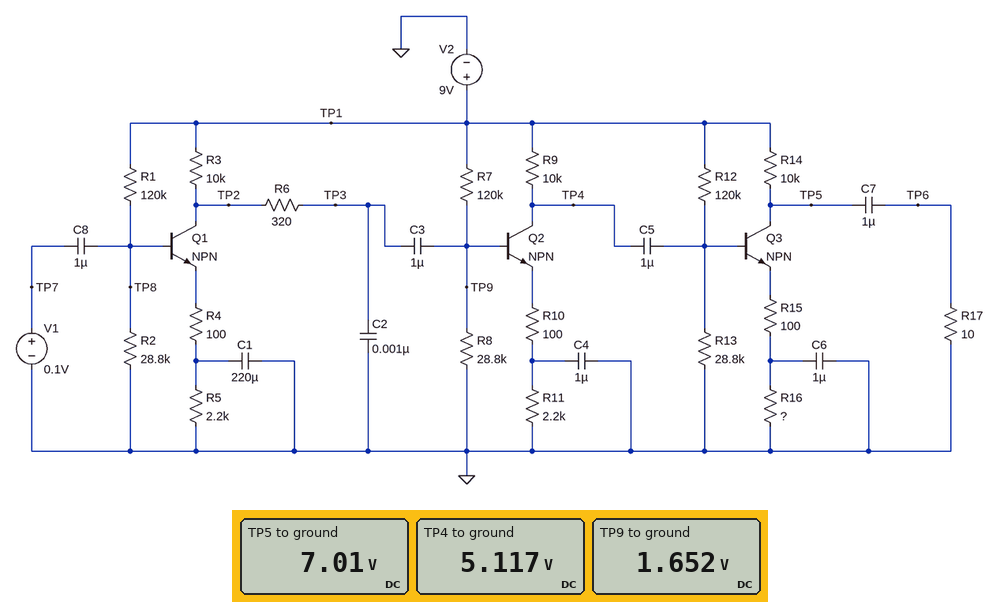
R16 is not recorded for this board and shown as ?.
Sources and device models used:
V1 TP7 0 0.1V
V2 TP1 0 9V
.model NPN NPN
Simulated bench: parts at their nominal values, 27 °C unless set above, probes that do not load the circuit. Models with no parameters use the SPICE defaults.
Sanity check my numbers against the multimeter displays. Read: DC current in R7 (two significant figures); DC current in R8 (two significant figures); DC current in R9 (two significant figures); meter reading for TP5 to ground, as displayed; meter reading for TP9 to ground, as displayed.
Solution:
61 µA
57 µA
390 µA
7.01 V
1.652 V
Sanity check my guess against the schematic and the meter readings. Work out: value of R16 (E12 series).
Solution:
4.7 kΩ
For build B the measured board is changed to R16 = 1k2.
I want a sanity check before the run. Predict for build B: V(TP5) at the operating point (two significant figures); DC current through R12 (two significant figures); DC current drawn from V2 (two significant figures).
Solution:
2.7 V
62 µA
1.6 mA
